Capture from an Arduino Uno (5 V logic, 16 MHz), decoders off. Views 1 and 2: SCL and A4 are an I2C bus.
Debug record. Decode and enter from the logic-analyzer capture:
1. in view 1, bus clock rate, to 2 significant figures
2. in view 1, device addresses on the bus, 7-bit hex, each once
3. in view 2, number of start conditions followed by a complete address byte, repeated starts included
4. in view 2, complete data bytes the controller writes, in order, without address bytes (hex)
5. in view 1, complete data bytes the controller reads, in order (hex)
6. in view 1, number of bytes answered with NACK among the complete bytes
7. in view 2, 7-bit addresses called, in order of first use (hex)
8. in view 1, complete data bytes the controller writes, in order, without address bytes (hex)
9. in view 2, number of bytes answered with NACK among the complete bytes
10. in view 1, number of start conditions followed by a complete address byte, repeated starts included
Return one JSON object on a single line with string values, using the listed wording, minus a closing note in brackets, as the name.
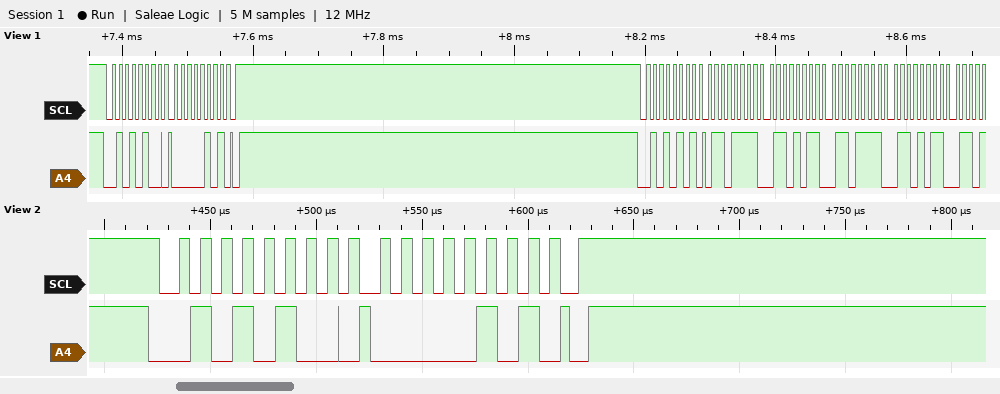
{"in view 1, bus clock rate, to 2 significant figures": "100 kHz", "in view 1, device addresses on the bus, 7-bit hex, each once": "0x2A", "in view 2, number of start conditions followed by a complete address byte, repeated starts included": "1", "in view 2, complete data bytes the controller writes, in order, without address bytes": "05", "in view 1, complete data bytes the controller reads, in order": "6F 6B 6F 6B", "in view 1, number of bytes answered with NACK among the complete bytes": "0", "in view 2, 7-bit addresses called, in order of first use": "0x2A", "in view 1, complete data bytes the controller writes, in order, without address bytes": "05", "in view 2, number of bytes answered with NACK among the complete bytes": "0", "in view 1, number of start conditions followed by a complete address byte, repeated starts included": "2"}
